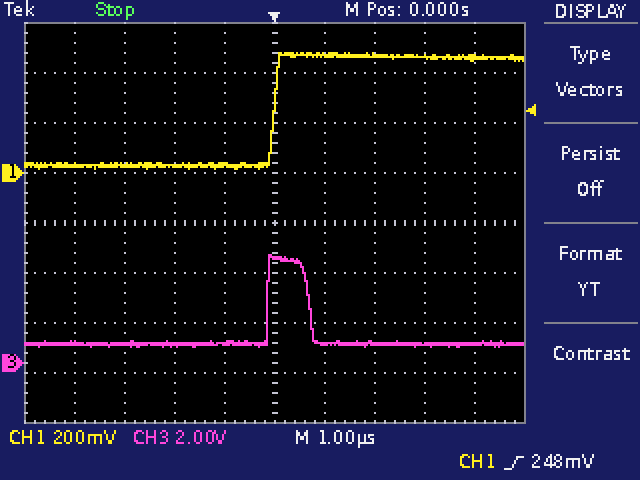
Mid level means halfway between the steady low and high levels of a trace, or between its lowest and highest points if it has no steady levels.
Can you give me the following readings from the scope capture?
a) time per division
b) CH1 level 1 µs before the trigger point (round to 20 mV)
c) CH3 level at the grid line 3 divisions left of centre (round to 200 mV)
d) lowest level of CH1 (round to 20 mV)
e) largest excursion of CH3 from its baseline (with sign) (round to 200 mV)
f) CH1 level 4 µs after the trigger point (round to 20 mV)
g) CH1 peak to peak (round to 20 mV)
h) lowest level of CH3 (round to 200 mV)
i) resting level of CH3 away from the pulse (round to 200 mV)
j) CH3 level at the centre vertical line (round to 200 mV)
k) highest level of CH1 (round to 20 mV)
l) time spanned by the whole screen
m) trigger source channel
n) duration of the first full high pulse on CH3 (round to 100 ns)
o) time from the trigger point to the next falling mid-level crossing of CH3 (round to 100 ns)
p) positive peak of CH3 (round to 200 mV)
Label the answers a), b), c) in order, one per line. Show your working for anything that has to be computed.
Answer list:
a) 1 µs
b) 40 mV
c) 800 mV
d) 20 mV
e) 4.4 V − (800 mV) = +3.6 V
f) 460 mV
g) 480 mV − (20 mV) = 460 mV
h) 600 mV
i) 800 mV
j) 4.2 V
k) 480 mV
l) 10 µs
m) CH1
n) 800 ns
o) 700 ns
p) 4.4 V
